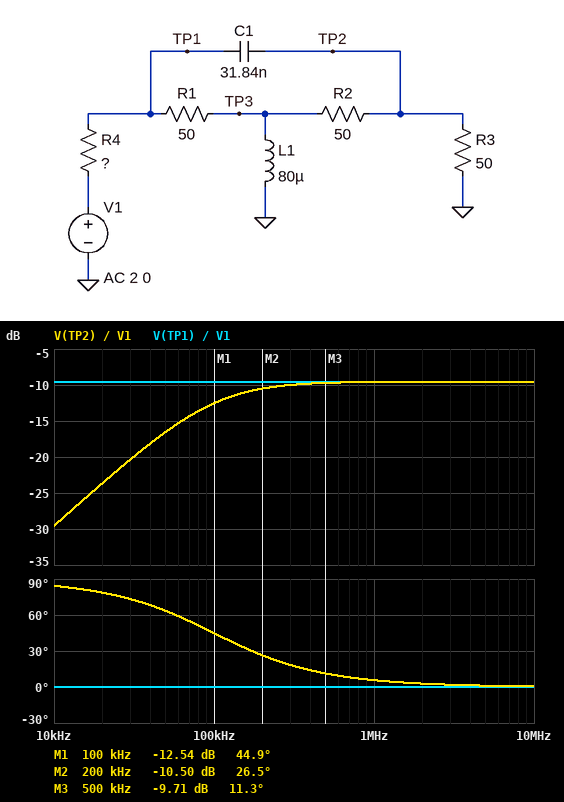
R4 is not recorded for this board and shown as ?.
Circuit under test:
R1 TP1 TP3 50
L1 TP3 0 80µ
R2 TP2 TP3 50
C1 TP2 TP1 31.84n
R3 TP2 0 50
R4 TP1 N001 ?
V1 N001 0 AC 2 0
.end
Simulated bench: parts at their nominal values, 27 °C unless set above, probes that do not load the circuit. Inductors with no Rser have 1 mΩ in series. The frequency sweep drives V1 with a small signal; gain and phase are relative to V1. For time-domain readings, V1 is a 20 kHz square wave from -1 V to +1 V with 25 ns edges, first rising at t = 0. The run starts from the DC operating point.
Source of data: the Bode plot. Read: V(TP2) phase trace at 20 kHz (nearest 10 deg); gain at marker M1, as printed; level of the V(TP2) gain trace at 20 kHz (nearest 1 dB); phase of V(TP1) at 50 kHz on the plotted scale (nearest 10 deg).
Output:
80 deg
-12.54 dB
-24 dB
0 deg
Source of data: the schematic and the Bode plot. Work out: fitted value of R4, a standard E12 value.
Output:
100 Ω
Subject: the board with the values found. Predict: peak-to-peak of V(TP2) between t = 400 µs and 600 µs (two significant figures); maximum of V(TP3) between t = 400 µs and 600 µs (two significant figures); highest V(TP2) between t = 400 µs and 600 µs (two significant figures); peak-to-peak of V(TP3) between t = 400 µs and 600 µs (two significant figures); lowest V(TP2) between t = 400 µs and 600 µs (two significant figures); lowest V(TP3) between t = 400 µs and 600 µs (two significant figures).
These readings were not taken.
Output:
1.3 V
660 mV
660 mV
1.3 V
-660 mV
-660 mV
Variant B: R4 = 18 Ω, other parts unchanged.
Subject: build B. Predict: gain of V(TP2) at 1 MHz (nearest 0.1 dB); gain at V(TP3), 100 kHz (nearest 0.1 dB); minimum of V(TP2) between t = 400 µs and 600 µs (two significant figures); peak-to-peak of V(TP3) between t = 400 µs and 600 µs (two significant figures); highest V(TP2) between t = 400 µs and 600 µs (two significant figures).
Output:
-2.7 dB
-5.7 dB
-1.5 V
2.9 V
1.5 V
